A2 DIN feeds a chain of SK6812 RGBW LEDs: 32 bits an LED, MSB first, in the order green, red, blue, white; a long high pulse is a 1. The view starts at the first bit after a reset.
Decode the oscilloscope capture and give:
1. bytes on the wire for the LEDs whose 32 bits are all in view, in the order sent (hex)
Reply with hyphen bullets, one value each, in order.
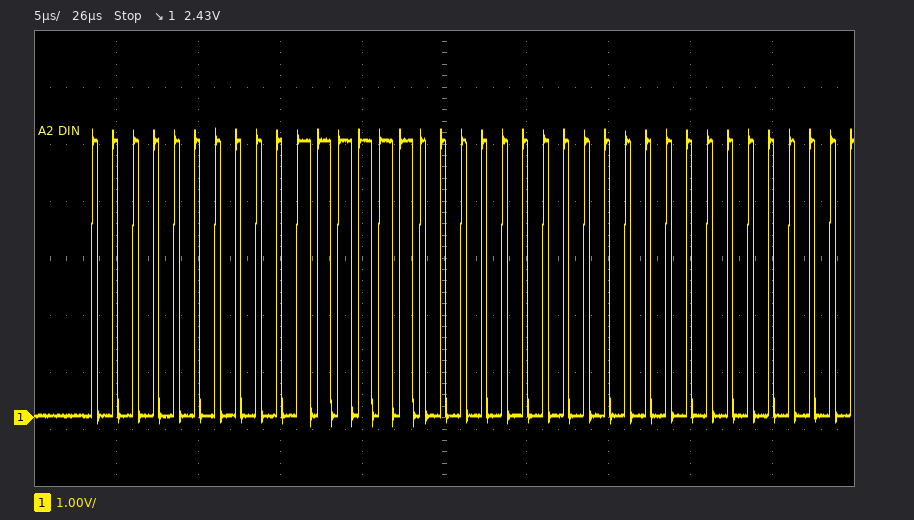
- 00 3F 00 00
